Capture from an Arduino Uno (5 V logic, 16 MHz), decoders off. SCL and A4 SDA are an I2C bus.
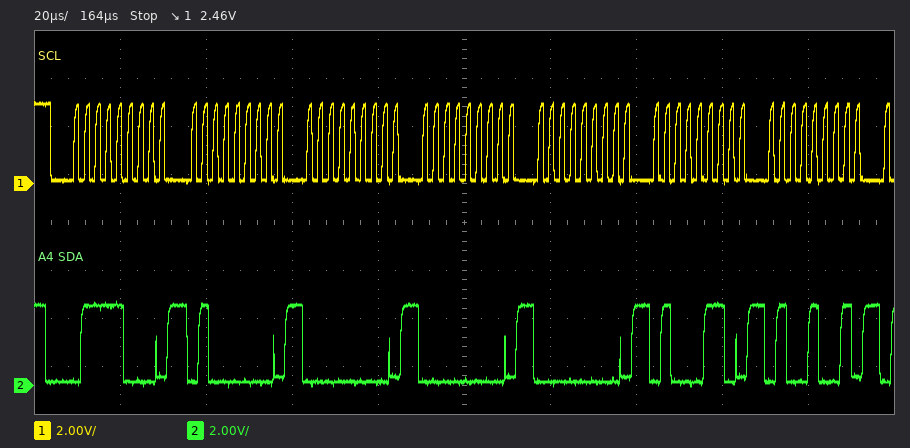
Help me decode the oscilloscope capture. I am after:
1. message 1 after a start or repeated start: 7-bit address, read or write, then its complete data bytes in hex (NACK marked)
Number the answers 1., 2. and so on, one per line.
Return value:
1. 0x3C write: 40 00 00 00 46 49
